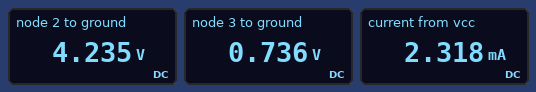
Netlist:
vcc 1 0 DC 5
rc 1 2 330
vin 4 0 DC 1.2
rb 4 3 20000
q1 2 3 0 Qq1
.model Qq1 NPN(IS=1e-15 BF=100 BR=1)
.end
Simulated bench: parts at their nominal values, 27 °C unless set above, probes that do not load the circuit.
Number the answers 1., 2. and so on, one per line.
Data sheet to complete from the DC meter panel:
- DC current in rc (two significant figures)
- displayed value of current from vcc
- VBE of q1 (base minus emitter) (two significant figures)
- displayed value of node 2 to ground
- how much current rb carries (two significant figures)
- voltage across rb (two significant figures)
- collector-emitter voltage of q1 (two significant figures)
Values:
1. 2.3 mA
2. 2.318 mA
3. 740 mV
4. 4.235 V
5. 23 µA
6. 460 mV
7. 4.2 V
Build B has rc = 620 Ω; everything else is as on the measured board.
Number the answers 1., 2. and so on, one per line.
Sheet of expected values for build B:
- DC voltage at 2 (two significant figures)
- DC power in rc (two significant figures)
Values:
1. 3.6 V
2. 3.3 mW
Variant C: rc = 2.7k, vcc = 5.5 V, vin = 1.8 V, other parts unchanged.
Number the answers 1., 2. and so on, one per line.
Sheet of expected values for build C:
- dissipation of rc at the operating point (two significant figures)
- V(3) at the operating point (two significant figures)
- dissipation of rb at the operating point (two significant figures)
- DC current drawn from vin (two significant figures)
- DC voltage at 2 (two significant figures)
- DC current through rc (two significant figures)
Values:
1. 11 mW
2. 730 mV
3. 57 µW
4. 53 µA
5. 110 mV
6. 2.0 mA
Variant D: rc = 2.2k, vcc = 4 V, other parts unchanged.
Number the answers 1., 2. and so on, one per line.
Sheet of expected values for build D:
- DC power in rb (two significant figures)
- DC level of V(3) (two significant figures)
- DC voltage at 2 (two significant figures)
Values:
1. 11 µW
2. 730 mV
3. 150 mV
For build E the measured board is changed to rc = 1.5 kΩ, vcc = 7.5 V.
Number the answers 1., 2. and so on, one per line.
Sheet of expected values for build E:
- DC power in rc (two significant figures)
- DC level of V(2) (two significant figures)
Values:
1. 8.1 mW
2. 4.0 V
